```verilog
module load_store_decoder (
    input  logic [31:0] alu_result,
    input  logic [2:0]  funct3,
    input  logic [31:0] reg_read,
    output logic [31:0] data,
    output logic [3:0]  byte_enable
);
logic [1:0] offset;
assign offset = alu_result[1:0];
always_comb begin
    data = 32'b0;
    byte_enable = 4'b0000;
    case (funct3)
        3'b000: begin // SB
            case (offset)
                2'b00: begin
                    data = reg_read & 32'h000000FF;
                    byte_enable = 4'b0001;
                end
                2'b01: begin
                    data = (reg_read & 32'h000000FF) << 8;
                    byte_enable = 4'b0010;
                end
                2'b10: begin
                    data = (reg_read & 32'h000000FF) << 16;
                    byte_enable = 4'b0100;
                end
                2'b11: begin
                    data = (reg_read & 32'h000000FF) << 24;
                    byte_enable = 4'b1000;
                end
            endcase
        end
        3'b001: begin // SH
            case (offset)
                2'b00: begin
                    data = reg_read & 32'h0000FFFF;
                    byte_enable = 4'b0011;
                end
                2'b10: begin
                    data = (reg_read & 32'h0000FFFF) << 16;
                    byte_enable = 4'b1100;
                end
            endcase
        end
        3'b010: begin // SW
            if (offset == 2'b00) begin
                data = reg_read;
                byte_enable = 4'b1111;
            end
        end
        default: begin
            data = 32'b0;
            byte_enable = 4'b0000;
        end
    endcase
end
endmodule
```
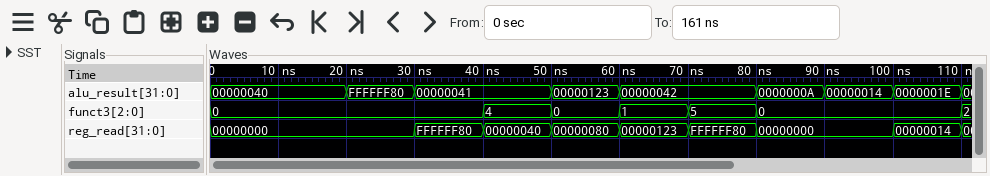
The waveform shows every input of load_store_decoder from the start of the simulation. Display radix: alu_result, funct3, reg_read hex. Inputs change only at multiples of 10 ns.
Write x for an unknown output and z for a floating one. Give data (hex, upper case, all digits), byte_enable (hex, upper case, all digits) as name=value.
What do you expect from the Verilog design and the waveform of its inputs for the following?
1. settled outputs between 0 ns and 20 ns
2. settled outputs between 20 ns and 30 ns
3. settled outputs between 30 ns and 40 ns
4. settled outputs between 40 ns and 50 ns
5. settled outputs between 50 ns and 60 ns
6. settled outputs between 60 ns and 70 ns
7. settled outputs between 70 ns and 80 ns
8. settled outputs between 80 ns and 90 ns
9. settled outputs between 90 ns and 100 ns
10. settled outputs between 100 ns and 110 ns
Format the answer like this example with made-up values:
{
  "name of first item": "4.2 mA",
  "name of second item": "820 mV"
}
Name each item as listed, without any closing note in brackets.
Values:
{
  "settled outputs between 0 ns and 20 ns": "data=00000000, byte_enable=1",
  "settled outputs between 20 ns and 30 ns": "data=00000000, byte_enable=1",
  "settled outputs between 30 ns and 40 ns": "data=00008000, byte_enable=2",
  "settled outputs between 40 ns and 50 ns": "data=00000000, byte_enable=0",
  "settled outputs between 50 ns and 60 ns": "data=80000000, byte_enable=8",
  "settled outputs between 60 ns and 70 ns": "data=01230000, byte_enable=C",
  "settled outputs between 70 ns and 80 ns": "data=00000000, byte_enable=0",
  "settled outputs between 80 ns and 90 ns": "data=00000000, byte_enable=4",
  "settled outputs between 90 ns and 100 ns": "data=00000000, byte_enable=1",
  "settled outputs between 100 ns and 110 ns": "data=00140000, byte_enable=4"
}
